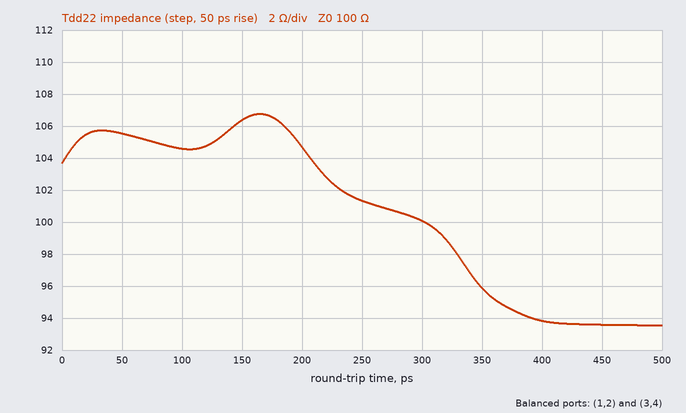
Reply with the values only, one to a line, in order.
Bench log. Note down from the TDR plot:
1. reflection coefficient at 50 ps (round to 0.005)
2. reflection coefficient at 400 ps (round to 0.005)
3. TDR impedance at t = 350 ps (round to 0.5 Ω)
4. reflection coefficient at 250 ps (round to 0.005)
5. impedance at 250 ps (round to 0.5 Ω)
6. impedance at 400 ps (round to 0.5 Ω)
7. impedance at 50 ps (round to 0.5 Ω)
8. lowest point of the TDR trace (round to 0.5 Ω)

+0.025
-0.030
96.0 Ω
+0.005
101.5 Ω
94.0 Ω
105.5 Ω
93.5 Ω
